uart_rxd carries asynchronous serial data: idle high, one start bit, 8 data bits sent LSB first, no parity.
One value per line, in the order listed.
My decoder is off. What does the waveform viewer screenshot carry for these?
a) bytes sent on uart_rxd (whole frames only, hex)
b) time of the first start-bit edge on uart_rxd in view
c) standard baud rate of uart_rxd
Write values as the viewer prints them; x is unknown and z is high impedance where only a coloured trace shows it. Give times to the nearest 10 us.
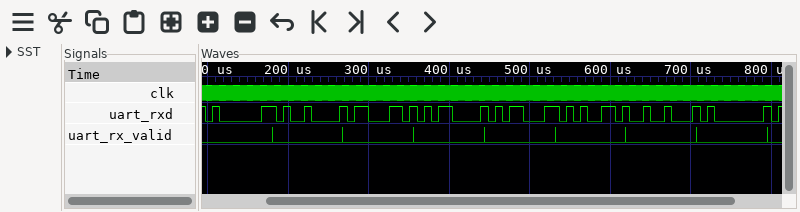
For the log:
81, 09, 63, 0D, 8D, 65, 12, 01
100 us
115200 baud
